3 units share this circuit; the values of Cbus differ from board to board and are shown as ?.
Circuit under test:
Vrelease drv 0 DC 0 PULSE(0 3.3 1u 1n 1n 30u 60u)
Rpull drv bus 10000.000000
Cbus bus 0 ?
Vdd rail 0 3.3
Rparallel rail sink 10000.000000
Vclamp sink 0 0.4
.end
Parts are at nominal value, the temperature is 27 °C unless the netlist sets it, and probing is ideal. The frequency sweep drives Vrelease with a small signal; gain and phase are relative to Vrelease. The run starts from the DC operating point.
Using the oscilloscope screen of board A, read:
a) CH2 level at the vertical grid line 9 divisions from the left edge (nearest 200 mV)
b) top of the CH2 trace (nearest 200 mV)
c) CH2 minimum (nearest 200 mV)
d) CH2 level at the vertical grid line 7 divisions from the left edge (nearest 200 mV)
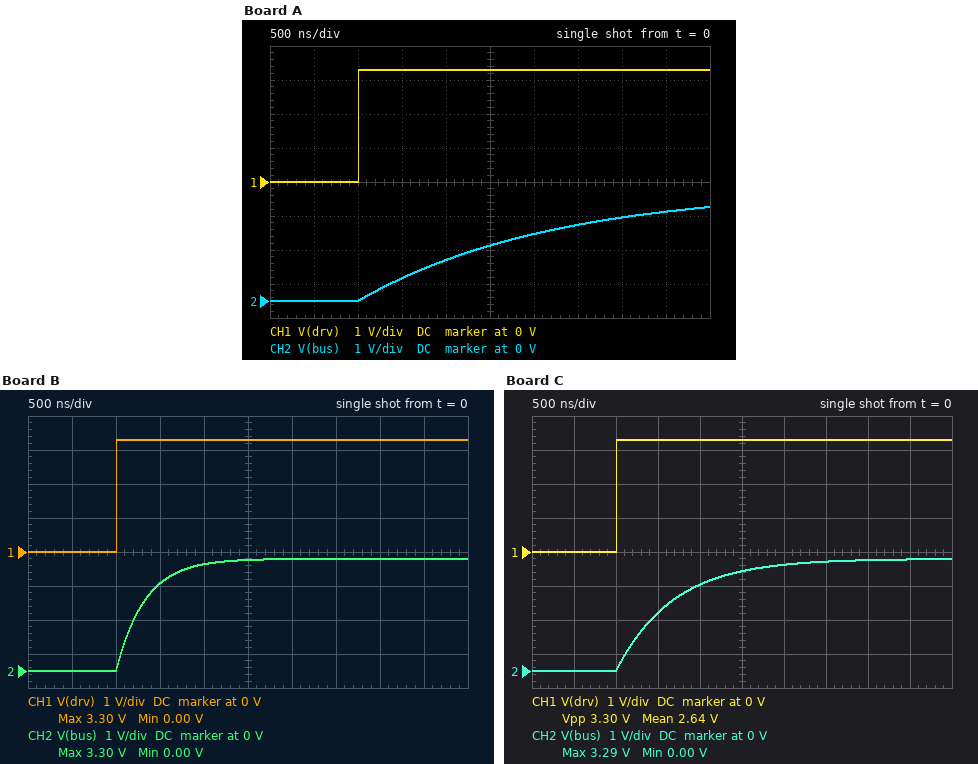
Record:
2.6 V
2.8 V
0 V
2.2 V
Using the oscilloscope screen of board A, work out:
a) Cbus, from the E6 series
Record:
220 pF
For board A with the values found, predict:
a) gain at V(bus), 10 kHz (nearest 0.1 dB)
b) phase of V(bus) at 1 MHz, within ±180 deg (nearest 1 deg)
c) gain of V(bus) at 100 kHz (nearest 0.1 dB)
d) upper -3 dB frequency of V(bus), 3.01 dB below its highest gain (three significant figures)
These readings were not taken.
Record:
-0.1 dB
-86 deg
-4.6 dB
72.3 kHz
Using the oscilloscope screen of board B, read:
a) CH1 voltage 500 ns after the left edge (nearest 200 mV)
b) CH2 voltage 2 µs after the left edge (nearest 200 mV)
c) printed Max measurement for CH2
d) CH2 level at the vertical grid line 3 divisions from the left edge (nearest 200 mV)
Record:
0 V
3.2 V
3.30 V
2.6 V
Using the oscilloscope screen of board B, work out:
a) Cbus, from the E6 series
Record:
33 pF
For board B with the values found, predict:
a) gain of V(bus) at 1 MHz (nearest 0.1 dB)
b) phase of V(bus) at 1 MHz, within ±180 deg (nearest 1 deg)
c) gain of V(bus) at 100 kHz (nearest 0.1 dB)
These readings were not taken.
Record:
-7.2 dB
-64 deg
-0.2 dB
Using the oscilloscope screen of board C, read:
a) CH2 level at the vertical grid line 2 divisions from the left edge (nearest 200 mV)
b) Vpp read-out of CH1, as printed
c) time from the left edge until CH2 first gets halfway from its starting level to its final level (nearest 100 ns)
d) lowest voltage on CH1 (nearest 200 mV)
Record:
0 V
3.30 V
1.5 µs
0 V
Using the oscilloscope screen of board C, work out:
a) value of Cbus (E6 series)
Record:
68 pF
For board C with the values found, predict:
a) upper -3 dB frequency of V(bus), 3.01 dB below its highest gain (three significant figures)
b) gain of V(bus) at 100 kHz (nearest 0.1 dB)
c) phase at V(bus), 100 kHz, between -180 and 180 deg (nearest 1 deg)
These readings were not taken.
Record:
234 kHz
-0.7 dB
-23 deg
